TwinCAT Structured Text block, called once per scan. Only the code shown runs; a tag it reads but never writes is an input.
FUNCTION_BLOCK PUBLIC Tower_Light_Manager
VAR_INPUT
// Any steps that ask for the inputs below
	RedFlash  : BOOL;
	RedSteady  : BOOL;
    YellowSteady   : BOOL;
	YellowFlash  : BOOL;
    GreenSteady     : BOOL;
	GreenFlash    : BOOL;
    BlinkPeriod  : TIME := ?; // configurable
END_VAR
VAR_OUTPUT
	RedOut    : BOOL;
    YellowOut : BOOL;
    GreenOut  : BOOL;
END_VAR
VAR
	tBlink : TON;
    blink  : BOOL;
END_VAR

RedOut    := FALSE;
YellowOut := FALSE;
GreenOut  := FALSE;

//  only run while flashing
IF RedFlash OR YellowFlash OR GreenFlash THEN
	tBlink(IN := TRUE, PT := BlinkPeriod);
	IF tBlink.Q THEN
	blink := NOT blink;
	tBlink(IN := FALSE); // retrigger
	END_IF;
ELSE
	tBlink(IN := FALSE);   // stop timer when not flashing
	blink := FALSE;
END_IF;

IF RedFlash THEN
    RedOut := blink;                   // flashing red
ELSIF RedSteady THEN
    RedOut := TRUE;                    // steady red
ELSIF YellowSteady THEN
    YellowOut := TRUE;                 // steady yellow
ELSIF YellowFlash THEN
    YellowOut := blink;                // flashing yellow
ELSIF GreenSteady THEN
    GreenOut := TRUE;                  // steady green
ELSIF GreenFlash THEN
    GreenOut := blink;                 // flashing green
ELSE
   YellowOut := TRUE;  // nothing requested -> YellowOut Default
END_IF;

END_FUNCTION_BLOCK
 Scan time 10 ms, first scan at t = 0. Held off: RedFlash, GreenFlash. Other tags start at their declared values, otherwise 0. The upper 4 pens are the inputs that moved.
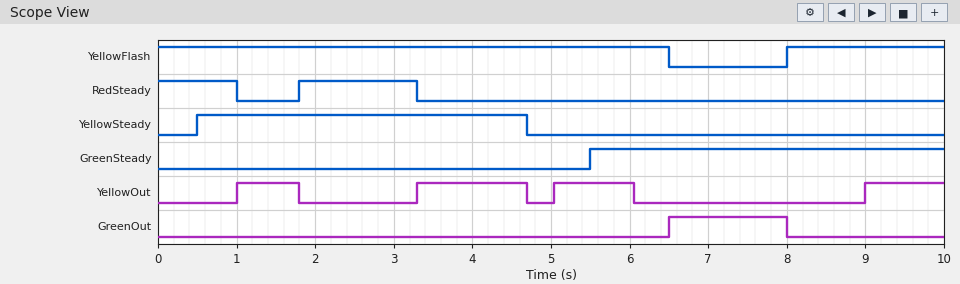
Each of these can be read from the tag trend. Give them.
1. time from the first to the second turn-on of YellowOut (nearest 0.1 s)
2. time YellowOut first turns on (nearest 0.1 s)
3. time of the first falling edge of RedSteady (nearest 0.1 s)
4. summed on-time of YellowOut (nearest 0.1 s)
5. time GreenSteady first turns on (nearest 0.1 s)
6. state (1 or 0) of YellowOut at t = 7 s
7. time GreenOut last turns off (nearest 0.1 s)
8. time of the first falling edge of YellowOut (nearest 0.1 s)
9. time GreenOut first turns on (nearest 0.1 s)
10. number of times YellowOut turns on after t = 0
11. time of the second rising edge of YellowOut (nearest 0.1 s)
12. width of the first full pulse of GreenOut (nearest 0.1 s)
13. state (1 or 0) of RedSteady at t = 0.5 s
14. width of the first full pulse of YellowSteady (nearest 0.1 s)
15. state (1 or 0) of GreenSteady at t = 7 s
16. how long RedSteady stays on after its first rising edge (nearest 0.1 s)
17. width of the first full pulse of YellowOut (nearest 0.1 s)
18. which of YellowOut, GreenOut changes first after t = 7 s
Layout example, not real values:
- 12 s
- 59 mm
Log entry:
- 2.3 s
- 1.0 s
- 1.0 s
- 4.2 s
- 5.5 s
- 0
- 8.0 s
- 1.8 s
- 6.5 s
- 4
- 3.3 s
- 1.5 s
- 1
- 4.2 s
- 1
- 1.5 s
- 0.8 s
- GreenOut
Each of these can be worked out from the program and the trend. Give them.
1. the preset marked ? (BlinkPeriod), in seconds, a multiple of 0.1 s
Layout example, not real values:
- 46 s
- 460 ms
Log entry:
- 1.0 s
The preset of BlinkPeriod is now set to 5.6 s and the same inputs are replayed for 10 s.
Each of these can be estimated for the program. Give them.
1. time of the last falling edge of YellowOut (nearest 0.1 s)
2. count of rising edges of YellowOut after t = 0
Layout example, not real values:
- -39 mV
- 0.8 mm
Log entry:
- 6.5 s
- 3
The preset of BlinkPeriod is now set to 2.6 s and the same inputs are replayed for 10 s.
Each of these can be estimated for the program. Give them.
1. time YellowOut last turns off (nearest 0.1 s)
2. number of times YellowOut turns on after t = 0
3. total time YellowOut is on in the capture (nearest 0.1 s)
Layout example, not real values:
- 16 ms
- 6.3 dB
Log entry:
- 5.2 s
- 2
- 2.7 s
